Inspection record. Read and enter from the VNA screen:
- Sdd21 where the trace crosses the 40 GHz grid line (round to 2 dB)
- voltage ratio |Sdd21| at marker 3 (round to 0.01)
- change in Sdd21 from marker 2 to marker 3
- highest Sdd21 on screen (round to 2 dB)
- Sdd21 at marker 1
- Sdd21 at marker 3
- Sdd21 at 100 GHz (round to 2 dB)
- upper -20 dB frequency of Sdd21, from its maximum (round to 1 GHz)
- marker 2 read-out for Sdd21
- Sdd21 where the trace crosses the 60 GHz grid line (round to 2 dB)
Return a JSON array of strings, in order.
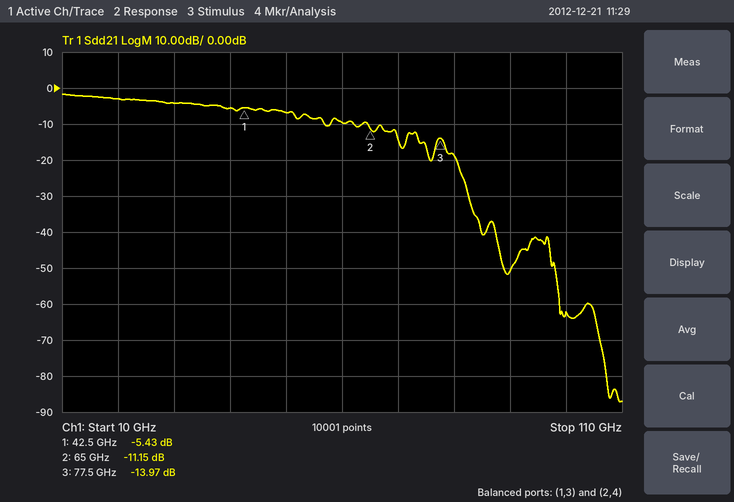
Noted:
["-6 dB", "0.20", "-2.82 dB", "-2 dB", "-5.43 dB", "-13.97 dB", "-62 dB", "81 GHz", "-11.15 dB", "-10 dB"]
